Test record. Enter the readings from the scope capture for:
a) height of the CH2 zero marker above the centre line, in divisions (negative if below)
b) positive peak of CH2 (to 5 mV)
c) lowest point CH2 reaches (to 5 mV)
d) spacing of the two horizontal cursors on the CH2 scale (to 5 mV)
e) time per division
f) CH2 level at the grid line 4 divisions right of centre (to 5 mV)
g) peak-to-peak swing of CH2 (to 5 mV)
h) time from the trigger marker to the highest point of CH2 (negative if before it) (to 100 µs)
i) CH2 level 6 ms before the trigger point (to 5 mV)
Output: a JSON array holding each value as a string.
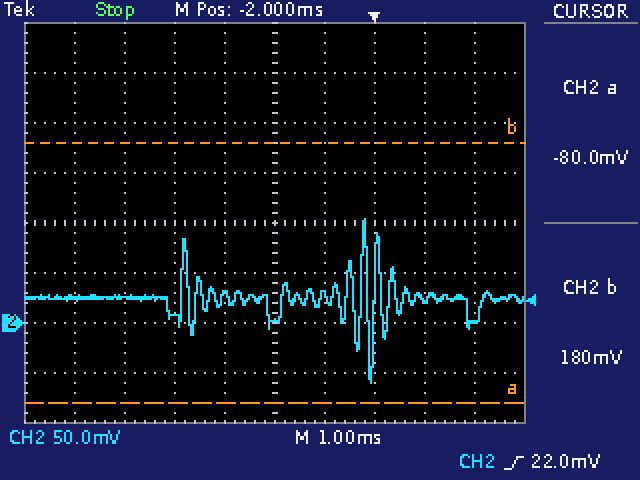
["-2.0 div", "105 mV", "-60 mV", "260 mV", "1 ms", "0 mV", "165 mV", "-200 µs", "25 mV"]
